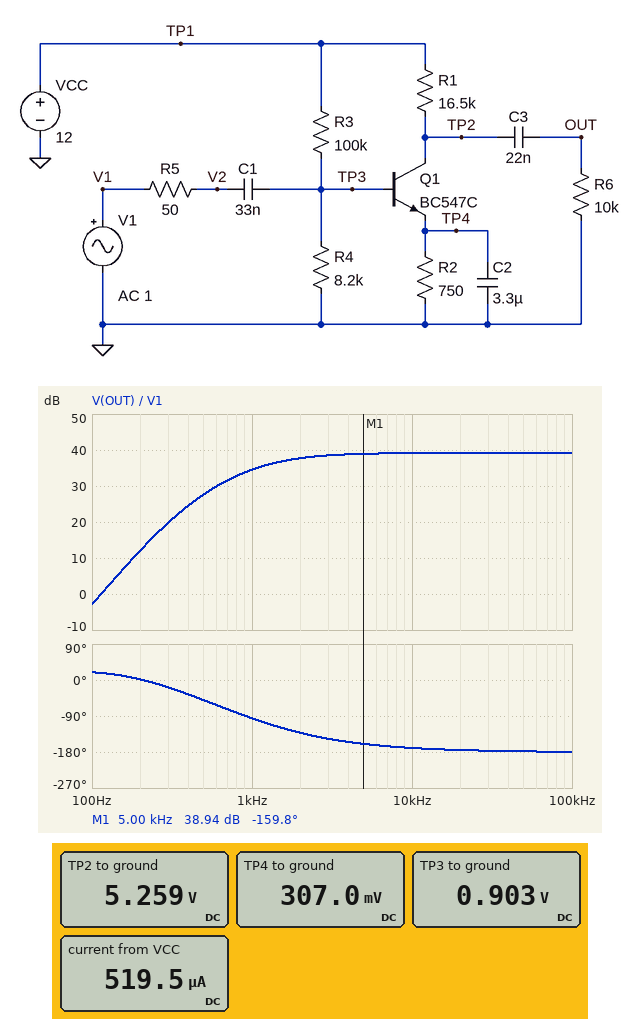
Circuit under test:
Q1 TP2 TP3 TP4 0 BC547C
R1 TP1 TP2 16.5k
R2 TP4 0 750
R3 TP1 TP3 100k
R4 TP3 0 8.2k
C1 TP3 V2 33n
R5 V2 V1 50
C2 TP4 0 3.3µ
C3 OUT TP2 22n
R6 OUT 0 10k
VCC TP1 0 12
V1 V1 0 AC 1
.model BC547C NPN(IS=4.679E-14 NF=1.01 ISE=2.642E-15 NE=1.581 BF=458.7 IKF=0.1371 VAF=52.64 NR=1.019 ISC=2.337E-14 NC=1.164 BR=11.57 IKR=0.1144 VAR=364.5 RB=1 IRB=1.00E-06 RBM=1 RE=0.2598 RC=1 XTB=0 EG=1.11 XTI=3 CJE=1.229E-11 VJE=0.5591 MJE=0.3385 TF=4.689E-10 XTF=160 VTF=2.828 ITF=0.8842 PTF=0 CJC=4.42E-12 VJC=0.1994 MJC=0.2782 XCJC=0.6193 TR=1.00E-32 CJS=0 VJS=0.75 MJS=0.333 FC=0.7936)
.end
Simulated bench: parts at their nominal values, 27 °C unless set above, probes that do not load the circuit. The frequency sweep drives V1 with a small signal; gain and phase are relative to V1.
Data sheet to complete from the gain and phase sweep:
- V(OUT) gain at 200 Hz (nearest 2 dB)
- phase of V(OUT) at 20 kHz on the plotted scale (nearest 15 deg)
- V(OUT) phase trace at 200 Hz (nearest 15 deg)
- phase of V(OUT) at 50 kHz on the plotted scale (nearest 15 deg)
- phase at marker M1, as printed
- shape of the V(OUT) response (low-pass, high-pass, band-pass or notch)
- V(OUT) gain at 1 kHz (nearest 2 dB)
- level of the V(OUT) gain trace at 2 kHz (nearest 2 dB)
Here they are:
12 dB
-180 deg
0 deg
-180 deg
-159.8 deg
high-pass
34 dB
38 dB
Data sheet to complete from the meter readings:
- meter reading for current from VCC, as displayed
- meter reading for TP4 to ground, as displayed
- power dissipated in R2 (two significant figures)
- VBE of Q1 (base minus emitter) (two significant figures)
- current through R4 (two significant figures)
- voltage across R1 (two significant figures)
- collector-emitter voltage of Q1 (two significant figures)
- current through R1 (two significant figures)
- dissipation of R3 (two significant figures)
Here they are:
519.5 µA
307.0 mV
130 µW
600 mV
110 µA
6.7 V
5.0 V
410 µA
1.2 mW
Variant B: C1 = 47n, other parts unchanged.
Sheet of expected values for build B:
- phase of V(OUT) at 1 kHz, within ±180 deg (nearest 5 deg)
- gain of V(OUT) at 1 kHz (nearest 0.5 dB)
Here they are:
-105 deg
35.5 dB
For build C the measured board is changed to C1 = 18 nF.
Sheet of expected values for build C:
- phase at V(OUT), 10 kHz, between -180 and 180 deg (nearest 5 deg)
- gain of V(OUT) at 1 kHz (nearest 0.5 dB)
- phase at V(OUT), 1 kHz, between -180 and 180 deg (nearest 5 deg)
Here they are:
-165 deg
32.0 dB
-80 deg
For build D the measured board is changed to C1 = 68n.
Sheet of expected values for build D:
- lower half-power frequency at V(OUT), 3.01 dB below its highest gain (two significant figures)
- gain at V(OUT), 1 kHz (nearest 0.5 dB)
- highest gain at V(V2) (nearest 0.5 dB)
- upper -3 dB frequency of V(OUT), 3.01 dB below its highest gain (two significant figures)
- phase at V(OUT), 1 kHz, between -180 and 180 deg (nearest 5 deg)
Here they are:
1.0 kHz
36.0 dB
0 dB
7.7 MHz
-110 deg
